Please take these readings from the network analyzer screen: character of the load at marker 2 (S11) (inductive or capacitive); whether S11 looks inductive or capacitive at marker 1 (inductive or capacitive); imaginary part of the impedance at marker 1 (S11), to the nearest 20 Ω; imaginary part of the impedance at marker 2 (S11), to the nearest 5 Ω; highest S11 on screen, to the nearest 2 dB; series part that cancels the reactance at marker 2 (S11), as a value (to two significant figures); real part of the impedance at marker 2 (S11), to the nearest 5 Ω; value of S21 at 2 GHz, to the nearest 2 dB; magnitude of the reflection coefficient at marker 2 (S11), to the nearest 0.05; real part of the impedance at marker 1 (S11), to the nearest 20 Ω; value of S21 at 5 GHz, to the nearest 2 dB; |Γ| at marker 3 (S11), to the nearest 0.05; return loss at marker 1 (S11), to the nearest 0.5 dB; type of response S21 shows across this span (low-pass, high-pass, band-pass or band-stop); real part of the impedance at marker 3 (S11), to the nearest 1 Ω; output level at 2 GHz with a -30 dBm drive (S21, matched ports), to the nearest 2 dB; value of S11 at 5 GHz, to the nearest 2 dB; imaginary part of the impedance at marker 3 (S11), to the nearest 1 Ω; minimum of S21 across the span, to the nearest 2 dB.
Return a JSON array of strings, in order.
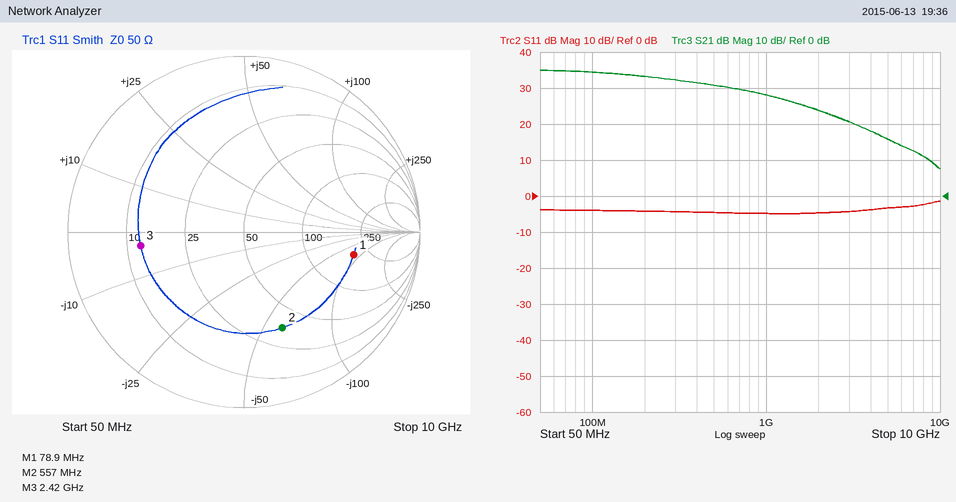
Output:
["capacitive", "capacitive", "-80 Ω", "-60 Ω", "-2 dB", "17 nH", "35 Ω", "24 dB", "0.60", "180 Ω", "16 dB", "0.60", "4.0 dB", "low-pass", "13 Ω", "-6 dBm", "-4 dB", "-3 Ω", "8 dB"]
